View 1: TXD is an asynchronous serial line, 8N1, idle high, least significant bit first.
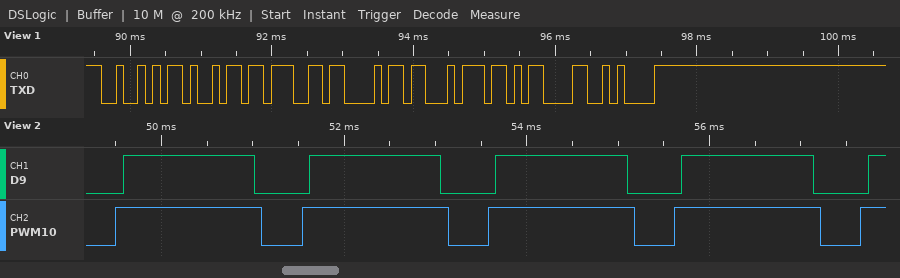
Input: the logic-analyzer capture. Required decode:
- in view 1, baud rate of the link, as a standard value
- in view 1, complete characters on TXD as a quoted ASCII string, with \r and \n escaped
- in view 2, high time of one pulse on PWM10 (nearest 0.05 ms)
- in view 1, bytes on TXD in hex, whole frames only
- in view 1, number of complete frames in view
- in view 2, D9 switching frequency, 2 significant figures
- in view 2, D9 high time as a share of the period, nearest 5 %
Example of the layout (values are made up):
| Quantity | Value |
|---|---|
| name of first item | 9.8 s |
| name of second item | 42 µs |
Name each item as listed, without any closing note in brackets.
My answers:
| Quantity | Value |
|---|---|
| in view 1, baud rate of the link, as a standard value | 9600 baud |
| in view 1, complete characters on TXD as a quoted ASCII string, with \r and \n escaped | "Right\r\n" |
| in view 2, high time of one pulse on PWM10 | 1.60 ms |
| in view 1, bytes on TXD in hex, whole frames only | 52 69 67 68 74 0D 0A |
| in view 1, number of complete frames in view | 7 |
| in view 2, D9 switching frequency, 2 significant figures | 490 Hz |
| in view 2, D9 high time as a share of the period, nearest 5 % | 70 % |
